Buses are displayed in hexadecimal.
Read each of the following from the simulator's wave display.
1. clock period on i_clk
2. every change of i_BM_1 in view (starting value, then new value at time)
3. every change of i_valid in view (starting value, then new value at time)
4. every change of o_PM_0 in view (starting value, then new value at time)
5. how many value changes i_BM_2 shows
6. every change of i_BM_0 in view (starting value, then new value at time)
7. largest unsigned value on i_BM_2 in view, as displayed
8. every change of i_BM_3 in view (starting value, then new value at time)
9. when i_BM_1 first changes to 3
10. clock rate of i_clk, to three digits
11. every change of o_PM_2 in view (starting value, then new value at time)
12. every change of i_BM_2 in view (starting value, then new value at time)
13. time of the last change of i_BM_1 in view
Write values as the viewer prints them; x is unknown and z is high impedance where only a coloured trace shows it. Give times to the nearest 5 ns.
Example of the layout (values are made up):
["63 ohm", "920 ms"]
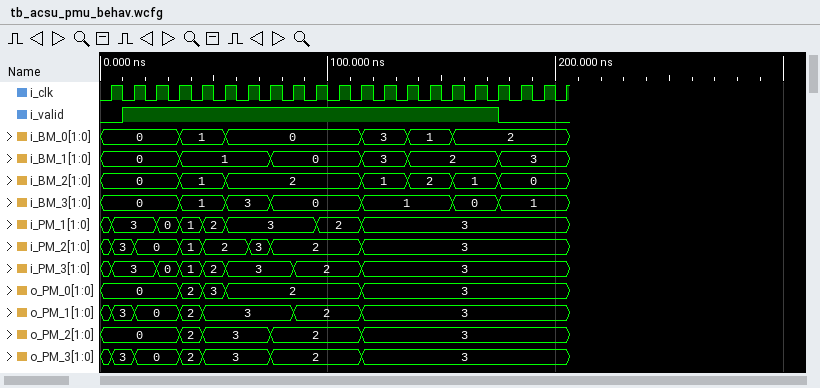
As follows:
["10 ns", "0, 1 at 35 ns, 0 at 75 ns, 3 at 115 ns, 2 at 135 ns, 3 at 175 ns", "0, 1 at 10 ns, 0 at 175 ns", "0, 2 at 35 ns, 3 at 45 ns, 2 at 55 ns, 3 at 115 ns", "6", "0, 1 at 35 ns, 0 at 55 ns, 3 at 115 ns, 1 at 135 ns, 2 at 155 ns", "2", "0, 1 at 35 ns, 3 at 55 ns, 0 at 75 ns, 1 at 115 ns, 0 at 155 ns, 1 at 175 ns", "115 ns", "100 MHz", "0, 2 at 35 ns, 3 at 45 ns, 2 at 75 ns, 3 at 115 ns", "0, 1 at 35 ns, 2 at 55 ns, 1 at 115 ns, 2 at 135 ns, 1 at 155 ns, 0 at 175 ns", "175 ns"]
